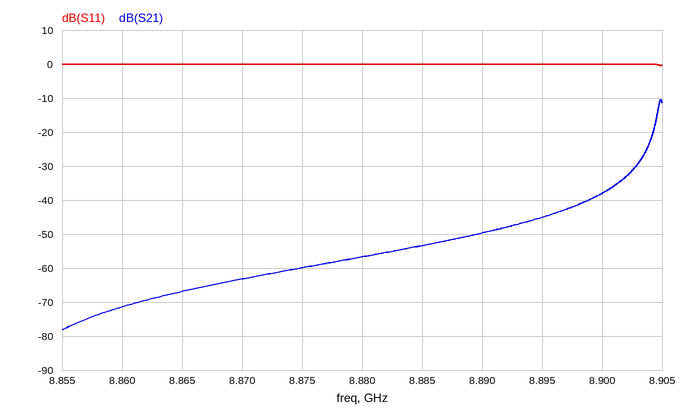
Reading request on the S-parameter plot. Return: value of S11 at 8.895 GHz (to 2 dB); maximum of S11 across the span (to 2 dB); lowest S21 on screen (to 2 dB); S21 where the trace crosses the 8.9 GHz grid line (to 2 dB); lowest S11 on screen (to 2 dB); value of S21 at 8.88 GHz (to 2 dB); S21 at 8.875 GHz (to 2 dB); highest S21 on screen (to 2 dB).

0 dB
0 dB
-78 dB
-38 dB
0 dB
-56 dB
-60 dB
-10 dB
